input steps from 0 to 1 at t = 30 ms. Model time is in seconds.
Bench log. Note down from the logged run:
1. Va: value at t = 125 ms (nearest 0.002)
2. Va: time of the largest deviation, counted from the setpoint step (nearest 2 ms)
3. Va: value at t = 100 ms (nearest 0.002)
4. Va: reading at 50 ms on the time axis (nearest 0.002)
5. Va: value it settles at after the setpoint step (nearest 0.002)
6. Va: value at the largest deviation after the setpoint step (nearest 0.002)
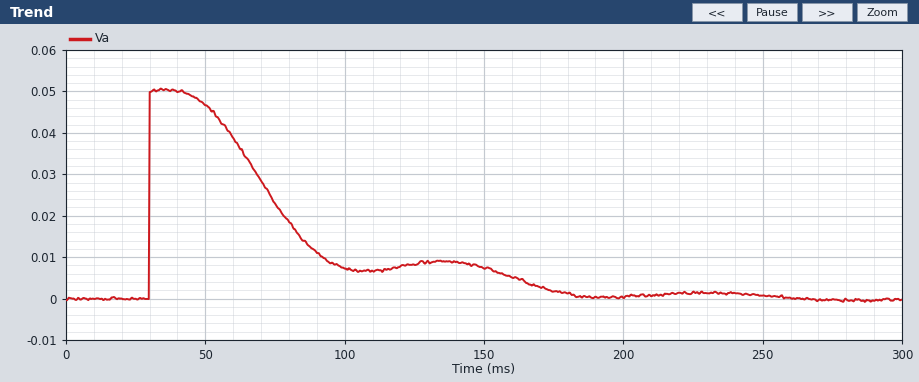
0.008
6 ms
0.008
0.046
0.000
0.050
